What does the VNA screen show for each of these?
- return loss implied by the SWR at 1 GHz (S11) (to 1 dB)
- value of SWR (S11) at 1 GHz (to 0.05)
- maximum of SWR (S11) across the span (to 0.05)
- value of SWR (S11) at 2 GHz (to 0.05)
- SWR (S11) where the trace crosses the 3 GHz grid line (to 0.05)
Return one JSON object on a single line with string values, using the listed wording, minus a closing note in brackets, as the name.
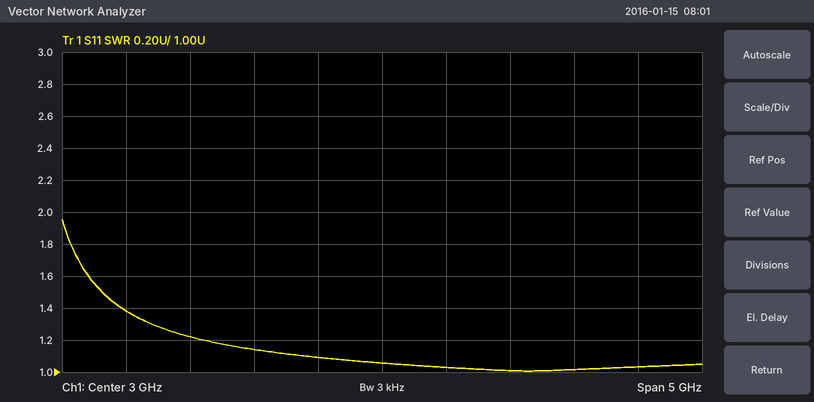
{"return loss implied by the SWR at 1 GHz (S11)": "16 dB", "value of SWR (S11) at 1 GHz": "1.40", "maximum of SWR (S11) across the span": "1.95", "value of SWR (S11) at 2 GHz": "1.15", "SWR (S11) where the trace crosses the 3 GHz grid line": "1.05"}
